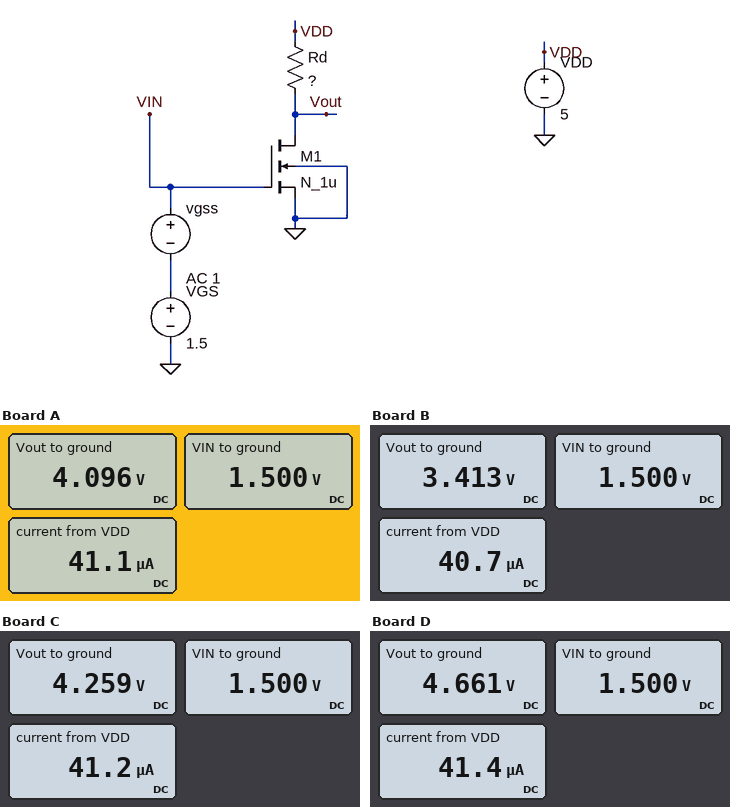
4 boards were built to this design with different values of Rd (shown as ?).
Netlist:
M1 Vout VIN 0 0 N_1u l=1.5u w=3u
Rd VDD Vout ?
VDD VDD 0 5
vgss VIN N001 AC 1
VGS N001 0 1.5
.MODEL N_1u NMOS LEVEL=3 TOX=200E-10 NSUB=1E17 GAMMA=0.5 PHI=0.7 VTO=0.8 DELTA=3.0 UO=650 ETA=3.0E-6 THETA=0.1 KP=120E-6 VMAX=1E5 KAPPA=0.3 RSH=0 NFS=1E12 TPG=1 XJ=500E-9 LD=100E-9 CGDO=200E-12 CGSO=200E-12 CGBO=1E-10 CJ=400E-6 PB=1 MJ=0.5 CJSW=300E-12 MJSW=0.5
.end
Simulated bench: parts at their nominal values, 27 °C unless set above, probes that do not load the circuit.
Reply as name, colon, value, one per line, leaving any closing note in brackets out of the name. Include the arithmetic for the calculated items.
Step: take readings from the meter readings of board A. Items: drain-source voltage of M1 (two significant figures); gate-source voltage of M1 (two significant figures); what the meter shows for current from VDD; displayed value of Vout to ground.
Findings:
drain-source voltage of M1: 4.096 V = 4.1 V
gate-source voltage of M1: 1.5 V = 1.5 V
what the meter shows for current from VDD: 41.1 µA
displayed value of Vout to ground: 4.096 V
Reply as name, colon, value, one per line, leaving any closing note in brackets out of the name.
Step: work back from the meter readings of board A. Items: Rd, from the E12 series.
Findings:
Rd, from the E12 series: 22 kΩ
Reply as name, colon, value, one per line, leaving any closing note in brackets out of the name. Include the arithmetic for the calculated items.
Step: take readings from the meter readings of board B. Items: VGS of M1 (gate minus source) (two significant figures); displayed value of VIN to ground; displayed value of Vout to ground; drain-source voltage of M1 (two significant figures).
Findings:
VGS of M1 (gate minus source): 1.5 V = 1.5 V
displayed value of VIN to ground: 1.500 V
displayed value of Vout to ground: 3.413 V
drain-source voltage of M1: 3.413 V = 3.4 V
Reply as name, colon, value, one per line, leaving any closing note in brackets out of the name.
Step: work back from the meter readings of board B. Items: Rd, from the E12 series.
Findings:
Rd, from the E12 series: 39 kΩ
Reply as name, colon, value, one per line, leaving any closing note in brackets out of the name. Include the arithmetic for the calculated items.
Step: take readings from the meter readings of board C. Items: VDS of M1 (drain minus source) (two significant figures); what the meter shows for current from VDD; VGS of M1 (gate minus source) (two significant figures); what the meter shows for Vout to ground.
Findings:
VDS of M1 (drain minus source): 4.259 V = 4.3 V
what the meter shows for current from VDD: 41.2 µA
VGS of M1 (gate minus source): 1.5 V = 1.5 V
what the meter shows for Vout to ground: 4.259 V
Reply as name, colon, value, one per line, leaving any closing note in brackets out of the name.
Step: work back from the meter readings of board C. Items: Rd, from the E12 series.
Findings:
Rd, from the E12 series: 18 kΩ
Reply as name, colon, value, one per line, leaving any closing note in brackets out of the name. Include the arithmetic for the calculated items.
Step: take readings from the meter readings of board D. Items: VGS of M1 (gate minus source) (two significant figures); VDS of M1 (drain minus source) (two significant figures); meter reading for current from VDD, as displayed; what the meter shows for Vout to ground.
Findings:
VGS of M1 (gate minus source): 1.5 V = 1.5 V
VDS of M1 (drain minus source): 4.661 V = 4.7 V
meter reading for current from VDD, as displayed: 41.4 µA
what the meter shows for Vout to ground: 4.661 V
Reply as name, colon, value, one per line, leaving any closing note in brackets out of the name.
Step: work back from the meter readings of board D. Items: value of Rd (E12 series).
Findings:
value of Rd: 8.2 kΩ
